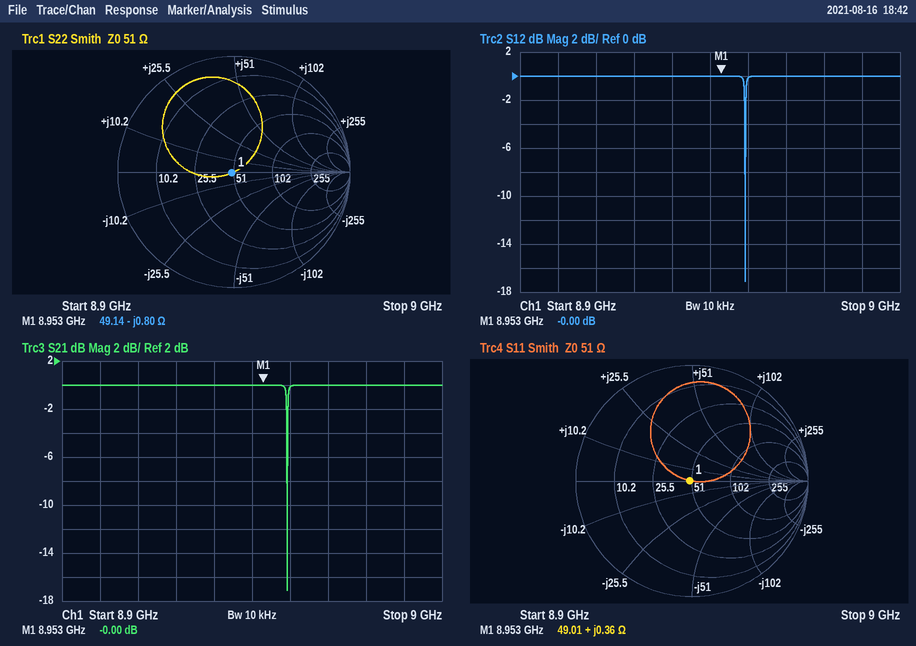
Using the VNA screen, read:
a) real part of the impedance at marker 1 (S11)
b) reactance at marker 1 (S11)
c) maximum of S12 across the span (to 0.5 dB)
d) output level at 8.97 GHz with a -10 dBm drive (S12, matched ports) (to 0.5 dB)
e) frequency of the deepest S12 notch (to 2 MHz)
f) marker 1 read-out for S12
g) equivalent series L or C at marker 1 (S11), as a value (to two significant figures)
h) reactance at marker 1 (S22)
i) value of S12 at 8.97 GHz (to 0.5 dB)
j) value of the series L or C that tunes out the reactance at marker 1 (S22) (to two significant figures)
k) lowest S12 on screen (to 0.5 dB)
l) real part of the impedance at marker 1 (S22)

49.01 Ω
+0.36 Ω
0.0 dB
-10.0 dBm
8.960 GHz
-0.00 dB
6.4 pH
-0.80 Ω
0.0 dB
14 pH
-17.0 dB
49.14 Ω
